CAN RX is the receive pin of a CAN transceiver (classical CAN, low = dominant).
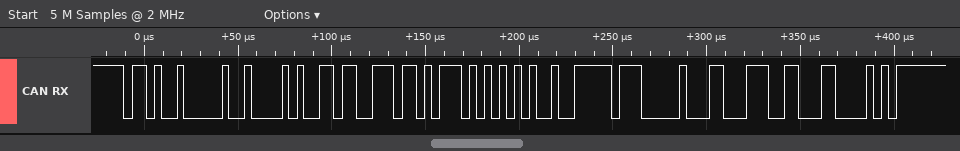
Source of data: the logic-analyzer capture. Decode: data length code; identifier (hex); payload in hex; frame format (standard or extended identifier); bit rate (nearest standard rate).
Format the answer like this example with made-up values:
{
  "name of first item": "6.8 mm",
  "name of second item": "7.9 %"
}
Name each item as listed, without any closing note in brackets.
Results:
{
  "data length code": "8",
  "identifier": "0x690",
  "payload in hex": "53 67 6B AA A4 FF 00 C7",
  "frame format": "standard",
  "bit rate": "250 kbit/s"
}
